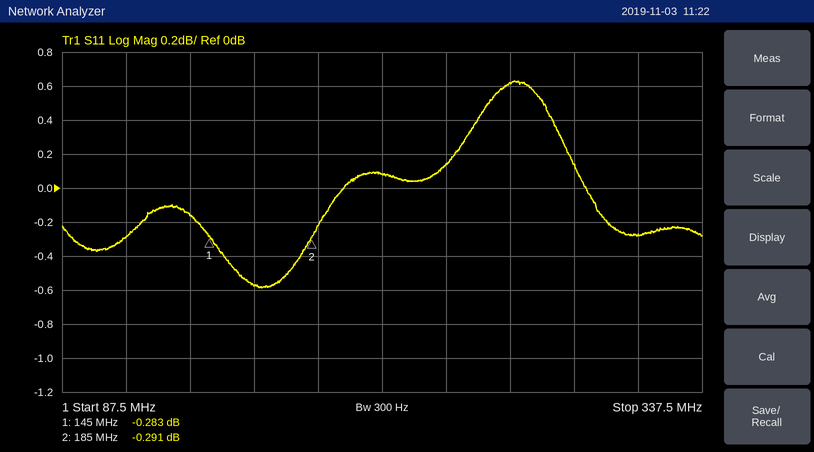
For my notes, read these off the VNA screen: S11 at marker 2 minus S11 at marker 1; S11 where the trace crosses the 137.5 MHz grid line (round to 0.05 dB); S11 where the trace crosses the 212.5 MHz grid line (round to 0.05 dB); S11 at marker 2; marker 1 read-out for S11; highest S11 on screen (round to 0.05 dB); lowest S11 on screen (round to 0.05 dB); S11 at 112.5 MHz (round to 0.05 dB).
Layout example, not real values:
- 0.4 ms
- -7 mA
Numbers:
- -0.008 dB
- -0.15 dB
- 0.10 dB
- -0.291 dB
- -0.283 dB
- 0.65 dB
- -0.60 dB
- -0.30 dB
